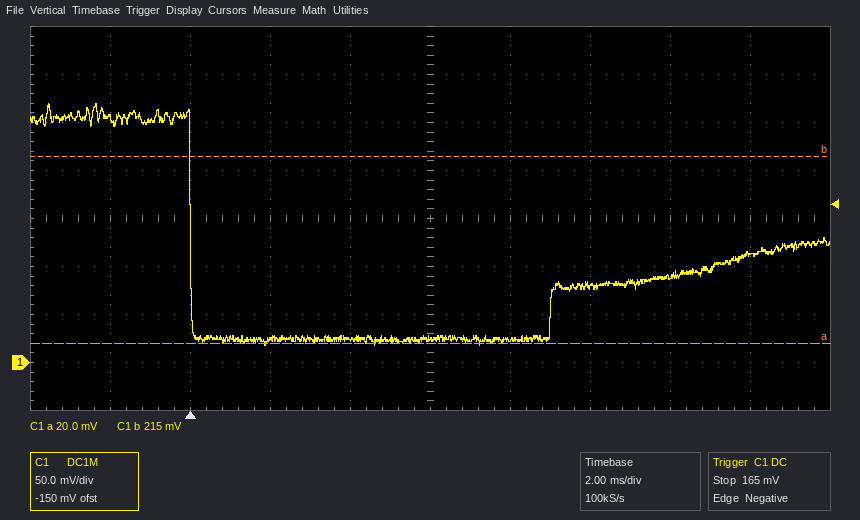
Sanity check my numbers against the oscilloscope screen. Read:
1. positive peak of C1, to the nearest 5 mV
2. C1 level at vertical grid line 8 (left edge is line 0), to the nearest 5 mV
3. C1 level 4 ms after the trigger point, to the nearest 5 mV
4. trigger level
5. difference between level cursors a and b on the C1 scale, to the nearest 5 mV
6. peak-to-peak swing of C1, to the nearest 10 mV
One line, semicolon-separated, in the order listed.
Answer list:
270 mV; 90 mV; 25 mV; 165 mV; 195 mV; 250 mV
